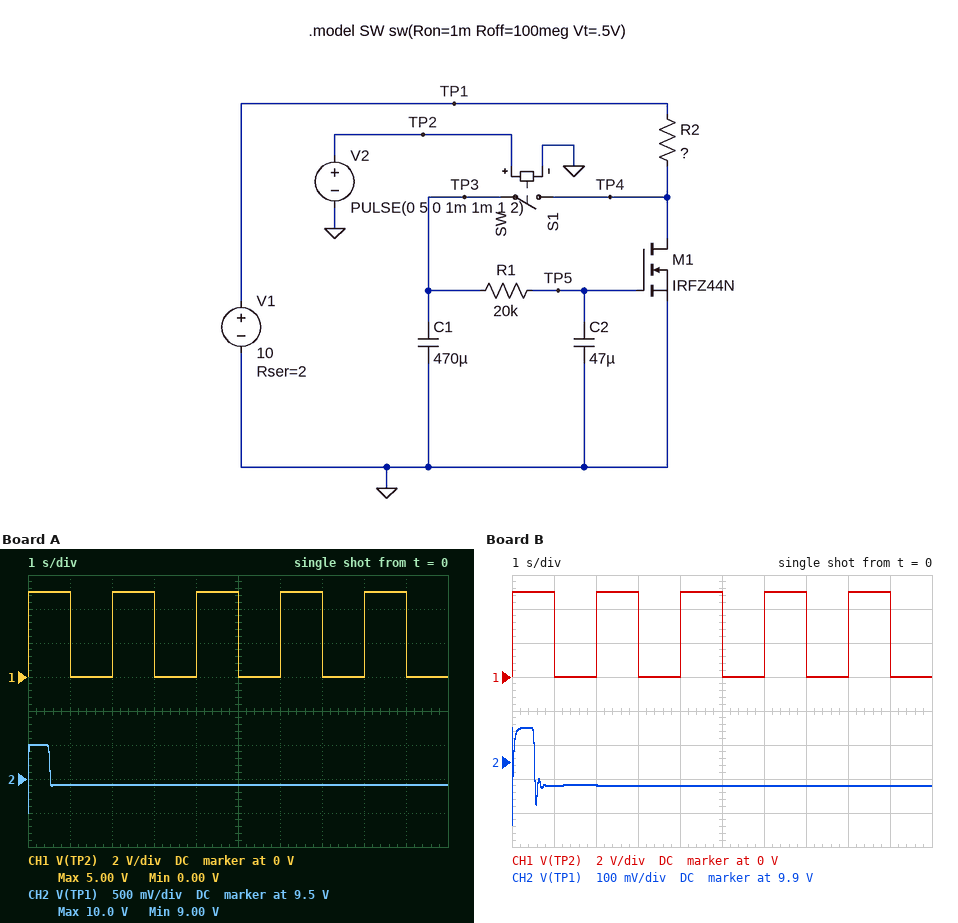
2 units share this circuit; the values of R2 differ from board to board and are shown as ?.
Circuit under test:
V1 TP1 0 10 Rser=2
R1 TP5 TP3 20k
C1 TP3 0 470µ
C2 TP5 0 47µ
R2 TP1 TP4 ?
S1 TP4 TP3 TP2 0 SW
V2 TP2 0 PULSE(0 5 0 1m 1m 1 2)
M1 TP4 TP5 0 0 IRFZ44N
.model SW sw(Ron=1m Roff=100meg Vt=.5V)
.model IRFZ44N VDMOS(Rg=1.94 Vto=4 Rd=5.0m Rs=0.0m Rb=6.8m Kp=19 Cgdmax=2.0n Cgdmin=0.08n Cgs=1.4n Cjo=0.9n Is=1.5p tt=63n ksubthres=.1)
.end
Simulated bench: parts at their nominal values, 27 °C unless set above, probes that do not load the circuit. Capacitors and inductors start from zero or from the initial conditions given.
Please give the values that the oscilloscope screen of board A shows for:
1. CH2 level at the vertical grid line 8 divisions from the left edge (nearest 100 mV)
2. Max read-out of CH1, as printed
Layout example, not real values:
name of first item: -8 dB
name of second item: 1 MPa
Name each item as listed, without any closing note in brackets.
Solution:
CH2 level at the vertical grid line 8 divisions from the left edge: 9.4 V
Max read-out of CH1, as printed: 5.00 V
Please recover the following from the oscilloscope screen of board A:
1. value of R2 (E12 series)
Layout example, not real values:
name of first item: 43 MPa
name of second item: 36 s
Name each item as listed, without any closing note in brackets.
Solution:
value of R2: 18 Ω
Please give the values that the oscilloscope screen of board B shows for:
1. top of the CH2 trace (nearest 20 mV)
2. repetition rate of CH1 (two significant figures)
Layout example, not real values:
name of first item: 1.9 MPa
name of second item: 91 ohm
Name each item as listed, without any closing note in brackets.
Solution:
top of the CH2 trace: 10.00 V
repetition rate of CH1: 500 mHz
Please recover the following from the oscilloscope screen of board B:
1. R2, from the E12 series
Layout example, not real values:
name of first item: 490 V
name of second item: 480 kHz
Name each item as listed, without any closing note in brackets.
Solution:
R2, from the E12 series: 68 Ω
